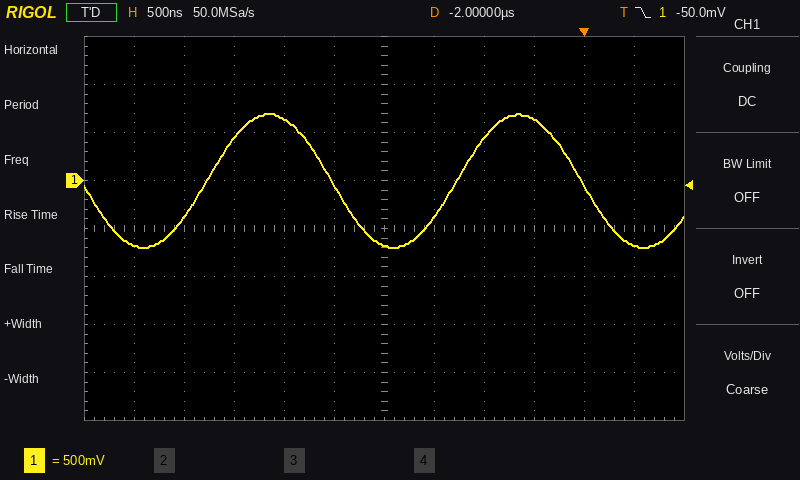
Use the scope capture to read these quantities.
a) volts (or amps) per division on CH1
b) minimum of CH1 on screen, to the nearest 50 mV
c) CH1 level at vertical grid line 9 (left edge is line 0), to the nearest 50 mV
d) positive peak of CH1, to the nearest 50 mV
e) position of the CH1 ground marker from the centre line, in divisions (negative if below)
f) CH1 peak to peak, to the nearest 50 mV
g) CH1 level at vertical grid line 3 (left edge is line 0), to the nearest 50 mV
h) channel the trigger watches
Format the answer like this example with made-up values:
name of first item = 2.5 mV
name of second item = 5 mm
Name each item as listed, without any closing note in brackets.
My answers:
volts (or amps) per division on CH1 = 500 mV
minimum of CH1 on screen, to the nearest 50 mV = -700 mV
CH1 level at vertical grid line 9 (left edge is line 0), to the nearest 50 mV = 650 mV
positive peak of CH1, to the nearest 50 mV = 700 mV
position of the CH1 ground marker from the centre line, in divisions = +1.0 div
CH1 peak to peak, to the nearest 50 mV = 1.40 V
CH1 level at vertical grid line 3 (left edge is line 0), to the nearest 50 mV = 450 mV
channel the trigger watches = CH1
